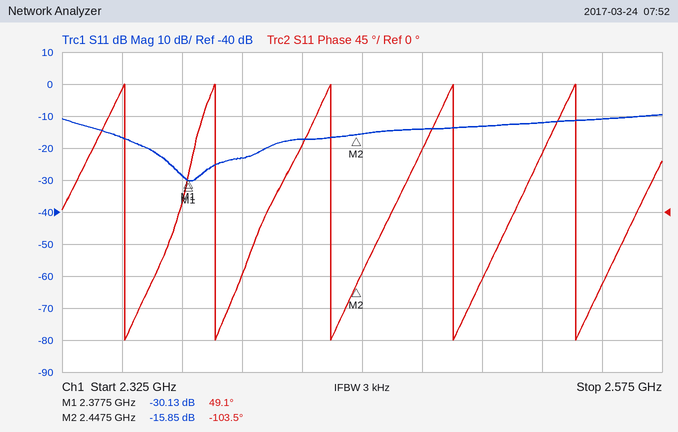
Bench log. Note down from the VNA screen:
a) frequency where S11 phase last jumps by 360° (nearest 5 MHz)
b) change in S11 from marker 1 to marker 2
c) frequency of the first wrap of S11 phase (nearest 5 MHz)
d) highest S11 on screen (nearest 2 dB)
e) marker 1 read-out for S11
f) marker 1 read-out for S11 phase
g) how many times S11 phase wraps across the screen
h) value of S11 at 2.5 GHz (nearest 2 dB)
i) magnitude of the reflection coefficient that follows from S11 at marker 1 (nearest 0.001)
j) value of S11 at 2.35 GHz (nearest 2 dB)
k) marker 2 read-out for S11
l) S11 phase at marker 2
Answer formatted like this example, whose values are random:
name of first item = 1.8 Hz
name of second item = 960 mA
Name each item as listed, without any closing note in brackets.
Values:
frequency where S11 phase last jumps by 360° = 2.540 GHz
change in S11 from marker 1 to marker 2 = 14.28 dB
frequency of the first wrap of S11 phase = 2.350 GHz
highest S11 on screen = -10 dB
marker 1 read-out for S11 = -30.13 dB
marker 1 read-out for S11 phase = 49.1°
how many times S11 phase wraps across the screen = 5
value of S11 at 2.5 GHz = -14 dB
magnitude of the reflection coefficient that follows from S11 at marker 1 = 0.031
value of S11 at 2.35 GHz = -16 dB
marker 2 read-out for S11 = -15.85 dB
S11 phase at marker 2 = -103.5°
